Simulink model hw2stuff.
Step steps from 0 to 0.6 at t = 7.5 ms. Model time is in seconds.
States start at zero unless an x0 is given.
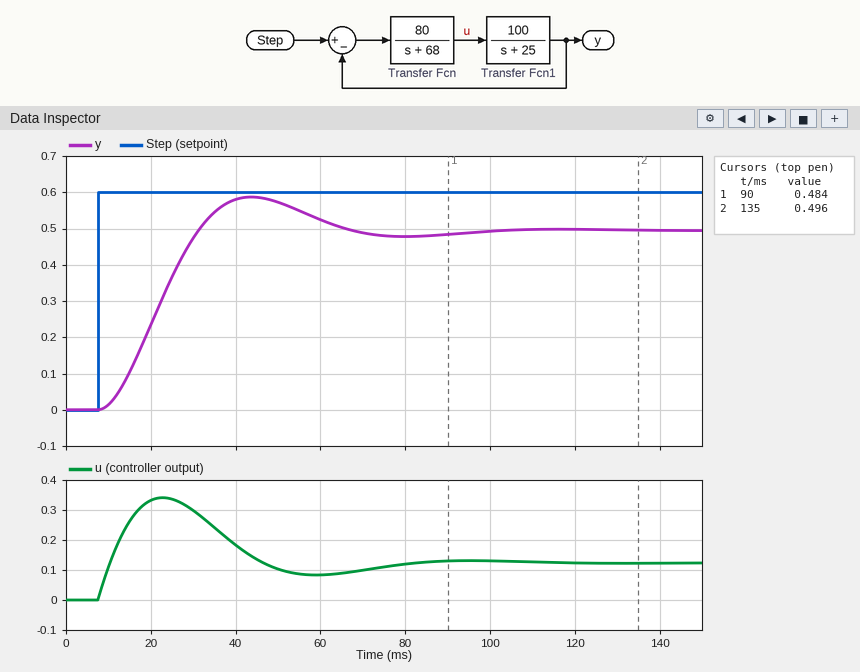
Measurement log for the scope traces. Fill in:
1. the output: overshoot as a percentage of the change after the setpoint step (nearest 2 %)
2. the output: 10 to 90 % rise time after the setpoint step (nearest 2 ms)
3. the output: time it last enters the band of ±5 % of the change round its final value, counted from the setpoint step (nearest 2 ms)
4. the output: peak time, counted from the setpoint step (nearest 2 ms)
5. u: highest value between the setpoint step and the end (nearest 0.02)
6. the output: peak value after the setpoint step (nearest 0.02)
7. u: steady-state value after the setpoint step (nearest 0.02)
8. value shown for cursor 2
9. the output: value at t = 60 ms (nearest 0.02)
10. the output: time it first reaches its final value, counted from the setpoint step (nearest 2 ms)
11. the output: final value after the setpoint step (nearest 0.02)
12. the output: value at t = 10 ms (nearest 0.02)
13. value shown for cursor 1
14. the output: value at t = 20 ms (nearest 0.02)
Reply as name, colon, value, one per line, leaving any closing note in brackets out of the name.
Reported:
the output: overshoot as a percentage of the change after the setpoint step: 18 %
the output: 10 to 90 % rise time after the setpoint step: 16 ms
the output: time it last enters the band of ±5 % of the change round its final value, counted from the setpoint step: 54 ms
the output: peak time, counted from the setpoint step: 36 ms
u: highest value between the setpoint step and the end: 0.34
the output: peak value after the setpoint step: 0.58
u: steady-state value after the setpoint step: 0.12
value shown for cursor 2: 0.496
the output: value at t = 60 ms: 0.52
the output: time it first reaches its final value, counted from the setpoint step: 24 ms
the output: final value after the setpoint step: 0.50
the output: value at t = 10 ms: 0.02
value shown for cursor 1: 0.484
the output: value at t = 20 ms: 0.24
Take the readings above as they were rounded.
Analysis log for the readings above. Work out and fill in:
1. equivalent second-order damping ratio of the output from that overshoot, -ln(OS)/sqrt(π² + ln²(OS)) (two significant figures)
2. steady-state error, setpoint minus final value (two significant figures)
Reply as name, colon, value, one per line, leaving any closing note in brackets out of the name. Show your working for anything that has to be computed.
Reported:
equivalent second-order damping ratio of the output from that overshoot, -ln(OS)/sqrt(π² + ln²(OS)): ln(0.18) = -1.715; 1.715 / sqrt(9.870 + 2.941) = 0.48
steady-state error, setpoint minus final value: 0.6 - 0.5 = 0.10
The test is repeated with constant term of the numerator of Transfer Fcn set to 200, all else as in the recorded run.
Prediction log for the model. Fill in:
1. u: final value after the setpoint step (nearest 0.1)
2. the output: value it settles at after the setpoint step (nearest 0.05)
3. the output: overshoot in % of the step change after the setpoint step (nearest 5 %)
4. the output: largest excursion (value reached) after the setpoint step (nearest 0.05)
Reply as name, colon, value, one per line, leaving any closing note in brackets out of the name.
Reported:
u: final value after the setpoint step: 0.1
the output: value it settles at after the setpoint step: 0.55
the output: overshoot in % of the step change after the setpoint step: 35 %
the output: largest excursion (value reached) after the setpoint step: 0.75
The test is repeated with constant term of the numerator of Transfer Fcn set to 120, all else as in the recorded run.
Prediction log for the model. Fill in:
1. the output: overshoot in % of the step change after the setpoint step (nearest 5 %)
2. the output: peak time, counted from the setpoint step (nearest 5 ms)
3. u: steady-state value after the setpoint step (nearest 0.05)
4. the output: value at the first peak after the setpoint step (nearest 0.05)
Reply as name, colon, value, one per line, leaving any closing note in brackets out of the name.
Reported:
the output: overshoot in % of the step change after the setpoint step: 25 %
the output: peak time, counted from the setpoint step: 30 ms
u: steady-state value after the setpoint step: 0.15
the output: value at the first peak after the setpoint step: 0.65
